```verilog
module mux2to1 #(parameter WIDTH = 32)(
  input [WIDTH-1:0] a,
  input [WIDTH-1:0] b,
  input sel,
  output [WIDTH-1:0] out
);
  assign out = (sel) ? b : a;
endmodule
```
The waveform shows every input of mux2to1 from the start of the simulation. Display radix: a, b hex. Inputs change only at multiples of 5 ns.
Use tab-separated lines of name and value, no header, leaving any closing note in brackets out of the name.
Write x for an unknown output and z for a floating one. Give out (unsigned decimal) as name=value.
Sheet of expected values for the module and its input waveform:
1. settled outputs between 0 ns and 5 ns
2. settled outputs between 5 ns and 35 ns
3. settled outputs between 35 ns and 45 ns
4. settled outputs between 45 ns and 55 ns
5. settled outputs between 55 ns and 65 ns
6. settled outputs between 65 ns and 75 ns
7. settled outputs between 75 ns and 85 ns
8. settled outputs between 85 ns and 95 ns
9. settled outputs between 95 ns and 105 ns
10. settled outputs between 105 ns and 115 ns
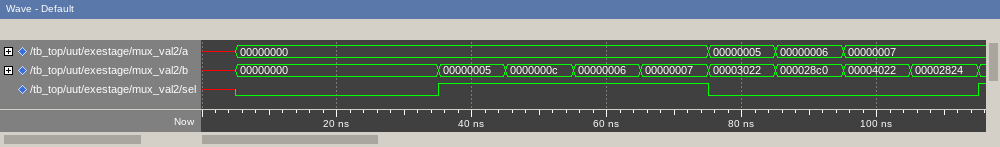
settled outputs between 0 ns and 5 ns	out=x
settled outputs between 5 ns and 35 ns	out=0
settled outputs between 35 ns and 45 ns	out=5
settled outputs between 45 ns and 55 ns	out=12
settled outputs between 55 ns and 65 ns	out=6
settled outputs between 65 ns and 75 ns	out=7
settled outputs between 75 ns and 85 ns	out=5
settled outputs between 85 ns and 95 ns	out=6
settled outputs between 95 ns and 105 ns	out=7
settled outputs between 105 ns and 115 ns	out=7
